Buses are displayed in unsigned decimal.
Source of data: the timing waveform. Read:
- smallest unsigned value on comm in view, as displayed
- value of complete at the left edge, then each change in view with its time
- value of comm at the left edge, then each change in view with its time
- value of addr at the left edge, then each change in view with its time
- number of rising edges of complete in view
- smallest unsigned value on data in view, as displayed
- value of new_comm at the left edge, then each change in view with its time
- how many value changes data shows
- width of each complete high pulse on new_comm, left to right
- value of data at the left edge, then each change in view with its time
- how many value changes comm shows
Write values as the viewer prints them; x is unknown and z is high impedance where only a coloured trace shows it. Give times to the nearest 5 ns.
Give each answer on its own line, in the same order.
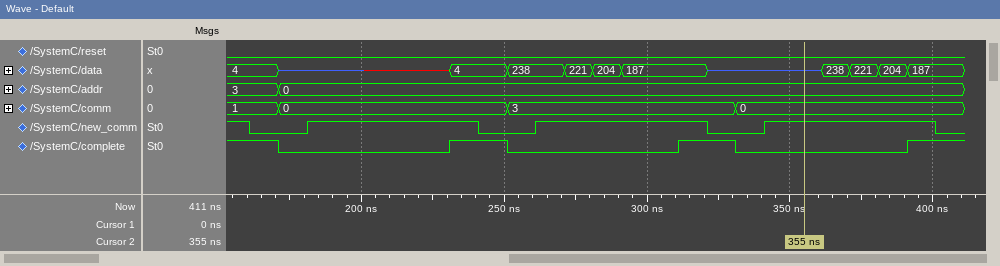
0
1, 0 at 170 ns, 1 at 230 ns, 0 at 250 ns, 1 at 310 ns, 0 at 330 ns, 1 at 390 ns
1, 0 at 170 ns, 3 at 250 ns, 0 at 330 ns
3, 0 at 170 ns
3
4
1, 0 at 160 ns, 1 at 180 ns, 0 at 240 ns, 1 at 260 ns, 0 at 320 ns, 1 at 340 ns, 0 at 400 ns
12
60 ns, 60 ns, 60 ns
4, z at 170 ns, x at 200 ns, 4 at 230 ns, 238 at 250 ns, 221 at 270 ns, 204 at 280 ns, 187 at 290 ns, z at 320 ns, 238 at 360 ns, 221 at 370 ns, 204 at 380 ns, 187 at 390 ns
3
